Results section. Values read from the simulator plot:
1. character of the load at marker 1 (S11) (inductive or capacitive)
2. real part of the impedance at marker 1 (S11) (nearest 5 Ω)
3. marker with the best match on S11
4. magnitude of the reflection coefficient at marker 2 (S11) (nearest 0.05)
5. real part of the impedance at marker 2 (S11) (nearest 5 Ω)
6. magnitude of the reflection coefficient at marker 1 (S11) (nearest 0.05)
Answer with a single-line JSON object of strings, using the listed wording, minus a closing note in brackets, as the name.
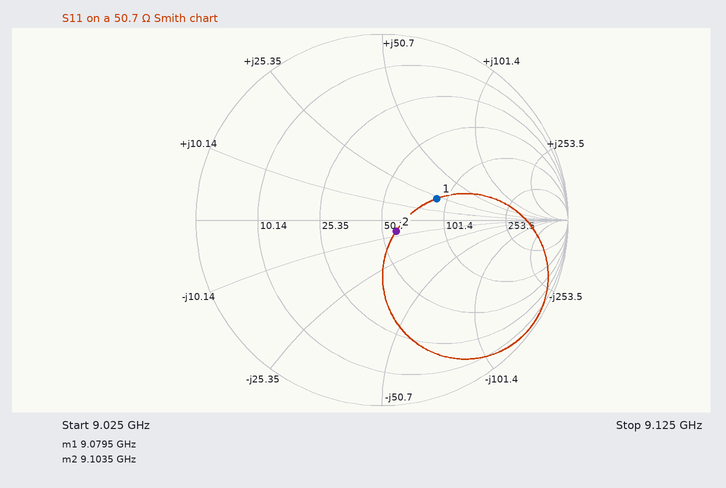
{"character of the load at marker 1 (S11)": "inductive", "real part of the impedance at marker 1 (S11)": "90 Ω", "marker with the best match on S11": "marker 2", "magnitude of the reflection coefficient at marker 2 (S11)": "0.10", "real part of the impedance at marker 2 (S11)": "60 Ω", "magnitude of the reflection coefficient at marker 1 (S11)": "0.30"}
